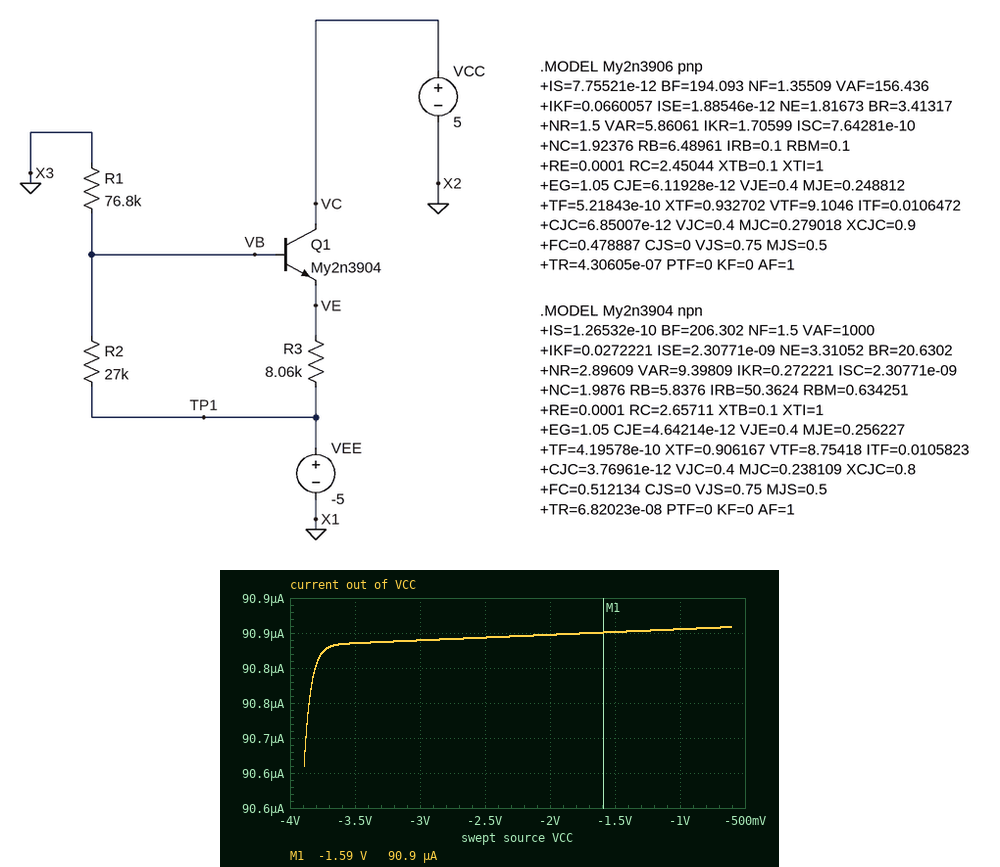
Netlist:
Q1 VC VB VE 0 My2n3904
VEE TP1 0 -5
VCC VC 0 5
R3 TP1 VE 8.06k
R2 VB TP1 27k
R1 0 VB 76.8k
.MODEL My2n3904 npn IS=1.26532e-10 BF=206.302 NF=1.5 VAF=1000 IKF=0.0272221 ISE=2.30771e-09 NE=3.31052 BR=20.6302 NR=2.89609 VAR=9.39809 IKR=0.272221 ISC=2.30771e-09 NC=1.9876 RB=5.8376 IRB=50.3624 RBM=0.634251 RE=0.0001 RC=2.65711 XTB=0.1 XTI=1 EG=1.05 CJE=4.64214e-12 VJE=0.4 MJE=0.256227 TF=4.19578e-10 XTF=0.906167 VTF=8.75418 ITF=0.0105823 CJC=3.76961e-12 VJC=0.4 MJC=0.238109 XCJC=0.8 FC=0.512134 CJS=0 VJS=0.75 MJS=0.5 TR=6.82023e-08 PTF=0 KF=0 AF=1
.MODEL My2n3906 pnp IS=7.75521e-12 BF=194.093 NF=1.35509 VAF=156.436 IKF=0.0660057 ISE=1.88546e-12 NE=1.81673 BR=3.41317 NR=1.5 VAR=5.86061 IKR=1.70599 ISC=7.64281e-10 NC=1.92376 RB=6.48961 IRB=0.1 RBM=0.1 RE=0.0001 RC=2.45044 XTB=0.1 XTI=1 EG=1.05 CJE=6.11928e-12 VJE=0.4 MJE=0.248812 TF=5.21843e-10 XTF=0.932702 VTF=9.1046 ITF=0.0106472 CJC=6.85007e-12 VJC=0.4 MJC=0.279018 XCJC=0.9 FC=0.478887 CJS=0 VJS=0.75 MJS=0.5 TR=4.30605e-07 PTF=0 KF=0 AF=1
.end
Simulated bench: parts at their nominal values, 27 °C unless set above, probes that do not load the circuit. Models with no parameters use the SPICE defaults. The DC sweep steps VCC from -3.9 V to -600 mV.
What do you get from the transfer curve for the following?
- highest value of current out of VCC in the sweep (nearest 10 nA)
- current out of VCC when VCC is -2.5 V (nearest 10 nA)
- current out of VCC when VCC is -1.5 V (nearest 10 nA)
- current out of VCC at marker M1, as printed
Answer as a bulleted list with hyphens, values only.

- 90.86 µA
- 90.84 µA
- 90.85 µA
- 90.9 µA
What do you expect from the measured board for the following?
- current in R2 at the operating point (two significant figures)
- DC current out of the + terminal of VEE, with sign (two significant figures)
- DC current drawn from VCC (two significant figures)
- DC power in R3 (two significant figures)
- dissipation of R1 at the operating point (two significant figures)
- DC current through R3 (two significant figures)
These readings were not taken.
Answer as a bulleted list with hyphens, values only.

- 47 µA
- -140 µA
- 91 µA
- 69 µW
- 180 µW
- 92 µA
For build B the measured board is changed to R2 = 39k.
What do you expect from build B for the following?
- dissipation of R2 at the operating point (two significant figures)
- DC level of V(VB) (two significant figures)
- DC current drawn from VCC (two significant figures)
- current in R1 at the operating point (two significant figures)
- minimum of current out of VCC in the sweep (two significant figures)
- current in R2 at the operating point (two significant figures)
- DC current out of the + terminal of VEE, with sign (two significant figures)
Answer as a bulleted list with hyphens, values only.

- 68 µW
- -3.4 V
- 130 µA
- 44 µA
- 110 µA
- 42 µA
- -180 µA
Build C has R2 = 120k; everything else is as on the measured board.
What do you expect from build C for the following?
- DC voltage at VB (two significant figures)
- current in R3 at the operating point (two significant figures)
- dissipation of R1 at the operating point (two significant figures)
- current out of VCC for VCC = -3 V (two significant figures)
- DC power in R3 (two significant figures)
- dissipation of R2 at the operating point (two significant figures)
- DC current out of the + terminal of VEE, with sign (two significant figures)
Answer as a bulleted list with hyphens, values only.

- -2.1 V
- 290 µA
- 58 µW
- 220 µA
- 670 µW
- 70 µW
- -310 µA
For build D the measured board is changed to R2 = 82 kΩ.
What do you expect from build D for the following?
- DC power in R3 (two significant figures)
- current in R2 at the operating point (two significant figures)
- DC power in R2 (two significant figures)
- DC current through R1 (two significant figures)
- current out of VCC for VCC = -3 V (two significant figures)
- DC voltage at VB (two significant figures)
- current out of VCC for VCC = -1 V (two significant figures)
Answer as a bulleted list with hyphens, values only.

- 450 µW
- 30 µA
- 74 µW
- 33 µA
- 220 µA
- -2.5 V
- 230 µA
